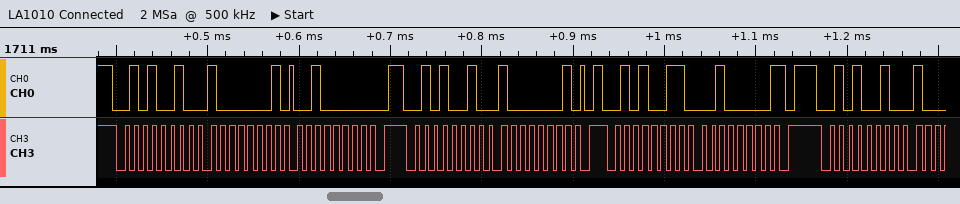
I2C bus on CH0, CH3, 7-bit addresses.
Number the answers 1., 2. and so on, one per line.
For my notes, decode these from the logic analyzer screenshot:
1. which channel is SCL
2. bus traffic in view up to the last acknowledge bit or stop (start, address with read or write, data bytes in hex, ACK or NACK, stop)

1. CH3
2. start, address 29 write ACK, 81 ACK, 20 ACK, stop, start, address 29 write ACK, 81 ACK, stop, start, address 29 read ACK, 20 NACK, stop, start, address 29 write ACK
